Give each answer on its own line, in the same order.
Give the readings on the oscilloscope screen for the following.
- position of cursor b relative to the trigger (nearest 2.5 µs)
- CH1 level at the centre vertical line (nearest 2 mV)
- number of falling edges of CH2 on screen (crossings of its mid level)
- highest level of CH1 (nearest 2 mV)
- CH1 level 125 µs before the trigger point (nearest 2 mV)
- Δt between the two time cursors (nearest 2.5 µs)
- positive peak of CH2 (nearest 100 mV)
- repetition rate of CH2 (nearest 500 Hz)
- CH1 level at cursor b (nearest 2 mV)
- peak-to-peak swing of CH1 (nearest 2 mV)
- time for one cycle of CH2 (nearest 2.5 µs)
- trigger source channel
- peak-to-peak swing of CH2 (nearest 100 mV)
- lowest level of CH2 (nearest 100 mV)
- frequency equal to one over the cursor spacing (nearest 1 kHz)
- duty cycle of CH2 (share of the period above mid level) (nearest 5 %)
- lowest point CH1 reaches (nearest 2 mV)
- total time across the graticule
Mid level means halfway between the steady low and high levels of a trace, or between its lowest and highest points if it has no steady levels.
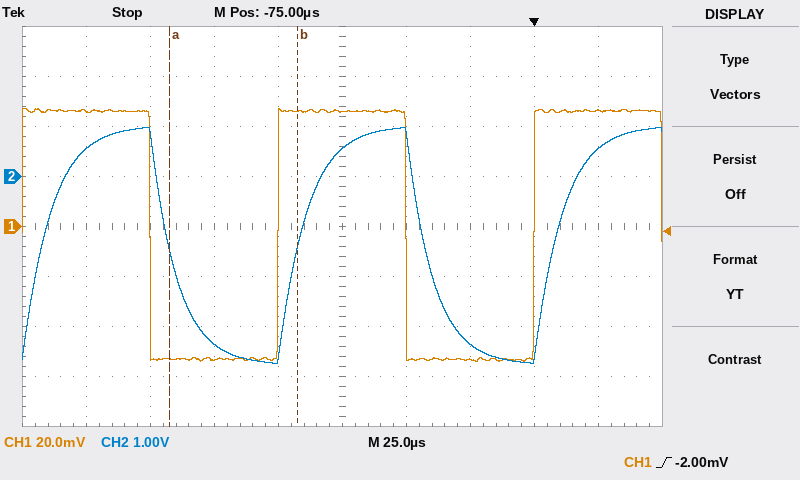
-92.5 µs
46 mV
2
48 mV
-54 mV
50.0 µs
1.0 V
10.0 kHz
46 mV
102 mV
100.0 µs
CH1
4.7 V
-3.7 V
20 kHz
50 %
-54 mV
250 µs
